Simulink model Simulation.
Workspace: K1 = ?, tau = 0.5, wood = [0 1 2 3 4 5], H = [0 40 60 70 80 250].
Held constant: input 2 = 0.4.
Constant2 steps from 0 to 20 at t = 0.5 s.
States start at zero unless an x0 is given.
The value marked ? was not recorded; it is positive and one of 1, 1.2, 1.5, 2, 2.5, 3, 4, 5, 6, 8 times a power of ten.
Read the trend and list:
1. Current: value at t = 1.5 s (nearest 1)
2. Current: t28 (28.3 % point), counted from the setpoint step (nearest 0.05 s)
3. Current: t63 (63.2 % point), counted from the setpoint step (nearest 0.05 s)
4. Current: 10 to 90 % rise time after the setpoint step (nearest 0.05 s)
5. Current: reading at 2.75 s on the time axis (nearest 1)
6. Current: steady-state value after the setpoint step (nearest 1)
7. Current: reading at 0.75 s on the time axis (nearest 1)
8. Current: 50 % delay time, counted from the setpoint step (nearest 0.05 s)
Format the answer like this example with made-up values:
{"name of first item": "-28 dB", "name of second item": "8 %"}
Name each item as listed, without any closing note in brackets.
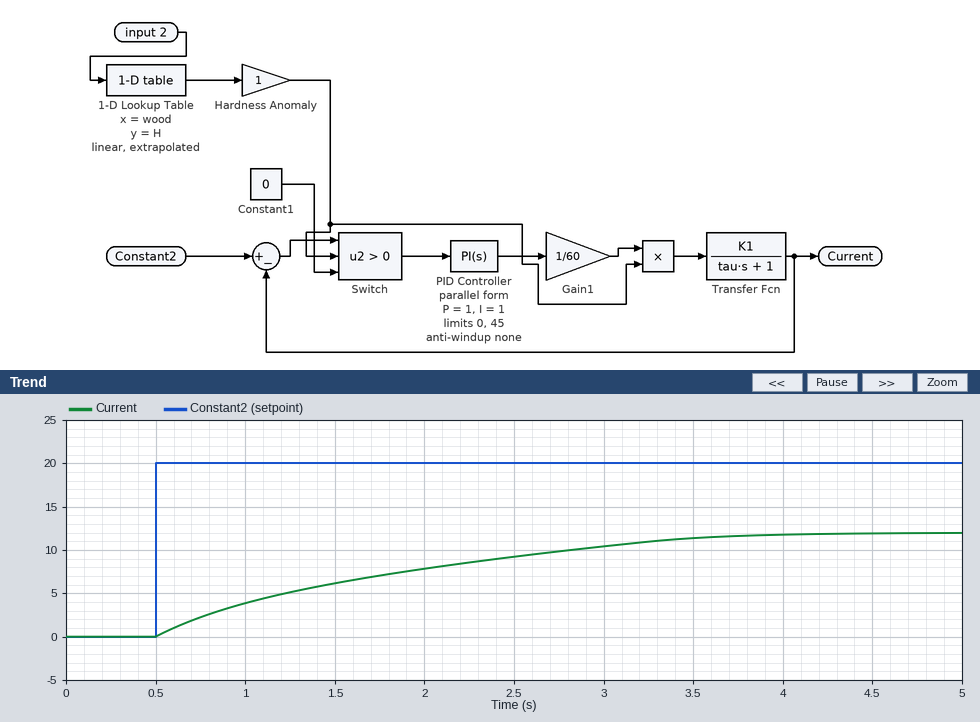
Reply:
{"Current: value at t = 1.5 s": "6", "Current: t28 (28.3 % point), counted from the setpoint step": "0.40 s", "Current: t63 (63.2 % point), counted from the setpoint step": "1.40 s", "Current: 10 to 90 % rise time after the setpoint step": "2.55 s", "Current: reading at 2.75 s on the time axis": "10", "Current: steady-state value after the setpoint step": "12", "Current: reading at 0.75 s on the time axis": "2", "Current: 50 % delay time, counted from the setpoint step": "0.95 s"}
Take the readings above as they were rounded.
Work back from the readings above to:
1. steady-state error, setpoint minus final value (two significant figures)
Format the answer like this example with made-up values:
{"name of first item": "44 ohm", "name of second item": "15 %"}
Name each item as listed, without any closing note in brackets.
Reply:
{"steady-state error, setpoint minus final value": "8.0"}
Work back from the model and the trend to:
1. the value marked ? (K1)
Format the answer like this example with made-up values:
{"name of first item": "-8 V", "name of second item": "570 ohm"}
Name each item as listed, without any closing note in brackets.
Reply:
{"the value marked ?": "1"}
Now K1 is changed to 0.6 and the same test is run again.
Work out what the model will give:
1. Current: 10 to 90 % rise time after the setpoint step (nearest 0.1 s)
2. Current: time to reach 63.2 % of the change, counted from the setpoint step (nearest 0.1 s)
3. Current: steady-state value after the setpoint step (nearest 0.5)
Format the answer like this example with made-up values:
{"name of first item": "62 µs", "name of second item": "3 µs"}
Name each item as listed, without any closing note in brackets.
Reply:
{"Current: 10 to 90 % rise time after the setpoint step": "2.0 s", "Current: time to reach 63.2 % of the change, counted from the setpoint step": "1.2 s", "Current: steady-state value after the setpoint step": "7.0"}
